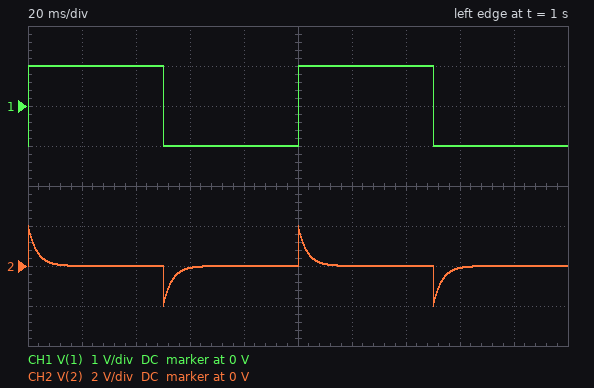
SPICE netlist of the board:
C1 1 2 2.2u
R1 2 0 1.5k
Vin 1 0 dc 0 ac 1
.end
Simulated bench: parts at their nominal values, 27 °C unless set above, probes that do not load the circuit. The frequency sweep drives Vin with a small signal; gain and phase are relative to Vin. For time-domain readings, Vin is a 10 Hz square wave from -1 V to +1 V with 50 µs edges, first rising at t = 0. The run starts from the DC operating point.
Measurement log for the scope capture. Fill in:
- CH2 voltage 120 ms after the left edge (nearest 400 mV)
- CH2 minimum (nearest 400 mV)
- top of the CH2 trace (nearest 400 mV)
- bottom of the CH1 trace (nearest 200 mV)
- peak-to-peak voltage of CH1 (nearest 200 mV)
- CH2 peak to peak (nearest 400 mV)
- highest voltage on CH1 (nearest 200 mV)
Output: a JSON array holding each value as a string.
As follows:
["0 V", "-2.0 V", "2.0 V", "-1.0 V", "2.0 V", "4.0 V", "1.0 V"]
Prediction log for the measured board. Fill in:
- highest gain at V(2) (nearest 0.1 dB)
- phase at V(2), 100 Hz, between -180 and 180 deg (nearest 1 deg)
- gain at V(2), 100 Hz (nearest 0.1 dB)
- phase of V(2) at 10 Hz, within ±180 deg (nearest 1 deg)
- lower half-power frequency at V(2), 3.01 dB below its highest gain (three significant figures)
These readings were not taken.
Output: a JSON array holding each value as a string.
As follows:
["0 dB", "26 deg", "-0.9 dB", "78 deg", "48.2 Hz"]
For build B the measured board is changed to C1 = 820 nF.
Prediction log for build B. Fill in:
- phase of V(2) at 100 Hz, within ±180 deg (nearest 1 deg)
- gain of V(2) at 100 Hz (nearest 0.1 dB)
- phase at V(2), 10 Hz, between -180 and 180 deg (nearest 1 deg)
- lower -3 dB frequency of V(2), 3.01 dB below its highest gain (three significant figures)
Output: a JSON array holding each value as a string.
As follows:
["52 deg", "-4.3 dB", "86 deg", "129 Hz"]
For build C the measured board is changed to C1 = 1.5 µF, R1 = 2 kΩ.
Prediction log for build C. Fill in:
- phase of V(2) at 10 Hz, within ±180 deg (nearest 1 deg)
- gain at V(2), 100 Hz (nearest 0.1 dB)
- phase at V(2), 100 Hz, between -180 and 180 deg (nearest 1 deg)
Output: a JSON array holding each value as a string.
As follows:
["79 deg", "-1.1 dB", "28 deg"]
